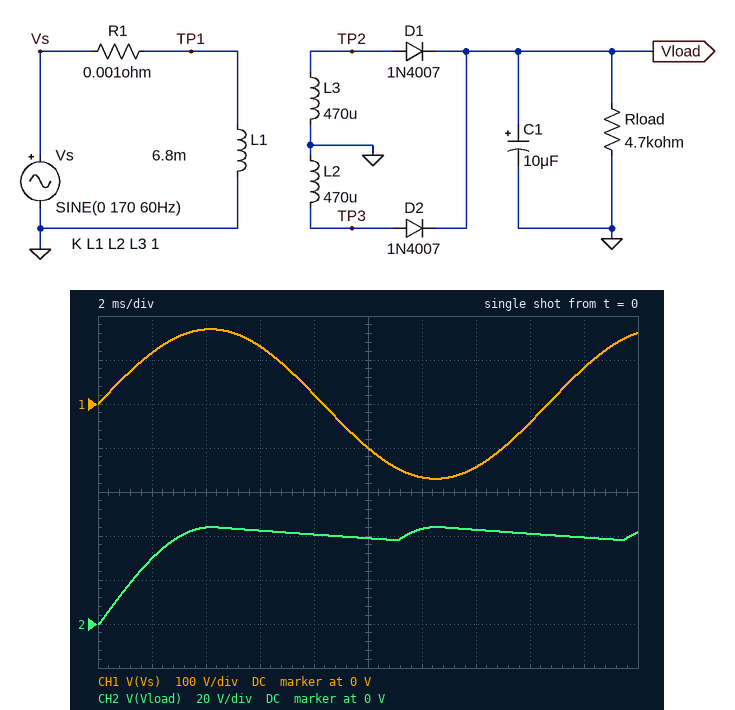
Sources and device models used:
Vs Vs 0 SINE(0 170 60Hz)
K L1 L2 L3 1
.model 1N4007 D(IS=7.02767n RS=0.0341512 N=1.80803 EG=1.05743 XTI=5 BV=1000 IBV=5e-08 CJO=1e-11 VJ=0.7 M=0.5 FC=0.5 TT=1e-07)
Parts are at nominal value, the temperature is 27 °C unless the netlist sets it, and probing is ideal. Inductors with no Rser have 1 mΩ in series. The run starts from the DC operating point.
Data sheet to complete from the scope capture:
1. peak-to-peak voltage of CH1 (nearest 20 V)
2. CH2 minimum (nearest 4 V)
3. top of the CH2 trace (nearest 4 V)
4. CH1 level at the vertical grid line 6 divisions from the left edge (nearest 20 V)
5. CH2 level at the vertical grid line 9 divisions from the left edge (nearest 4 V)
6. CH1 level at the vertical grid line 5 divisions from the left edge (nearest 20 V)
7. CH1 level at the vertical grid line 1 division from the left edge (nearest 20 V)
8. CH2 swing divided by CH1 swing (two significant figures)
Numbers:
340 V
0 V
44 V
-160 V
40 V
-100 V
120 V
0.13
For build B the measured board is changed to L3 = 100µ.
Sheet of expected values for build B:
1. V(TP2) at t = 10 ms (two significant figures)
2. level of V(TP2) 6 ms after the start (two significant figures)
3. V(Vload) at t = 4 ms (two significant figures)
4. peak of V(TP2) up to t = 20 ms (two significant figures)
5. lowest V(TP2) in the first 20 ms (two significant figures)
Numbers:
-12 V
16 V
20 V
21 V
-21 V
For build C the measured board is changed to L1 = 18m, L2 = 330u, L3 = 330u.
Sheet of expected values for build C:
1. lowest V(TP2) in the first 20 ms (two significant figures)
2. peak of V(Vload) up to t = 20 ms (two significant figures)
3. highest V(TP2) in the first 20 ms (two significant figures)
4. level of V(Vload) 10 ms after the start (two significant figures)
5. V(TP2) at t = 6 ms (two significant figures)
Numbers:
-23 V
22 V
23 V
20 V
18 V
